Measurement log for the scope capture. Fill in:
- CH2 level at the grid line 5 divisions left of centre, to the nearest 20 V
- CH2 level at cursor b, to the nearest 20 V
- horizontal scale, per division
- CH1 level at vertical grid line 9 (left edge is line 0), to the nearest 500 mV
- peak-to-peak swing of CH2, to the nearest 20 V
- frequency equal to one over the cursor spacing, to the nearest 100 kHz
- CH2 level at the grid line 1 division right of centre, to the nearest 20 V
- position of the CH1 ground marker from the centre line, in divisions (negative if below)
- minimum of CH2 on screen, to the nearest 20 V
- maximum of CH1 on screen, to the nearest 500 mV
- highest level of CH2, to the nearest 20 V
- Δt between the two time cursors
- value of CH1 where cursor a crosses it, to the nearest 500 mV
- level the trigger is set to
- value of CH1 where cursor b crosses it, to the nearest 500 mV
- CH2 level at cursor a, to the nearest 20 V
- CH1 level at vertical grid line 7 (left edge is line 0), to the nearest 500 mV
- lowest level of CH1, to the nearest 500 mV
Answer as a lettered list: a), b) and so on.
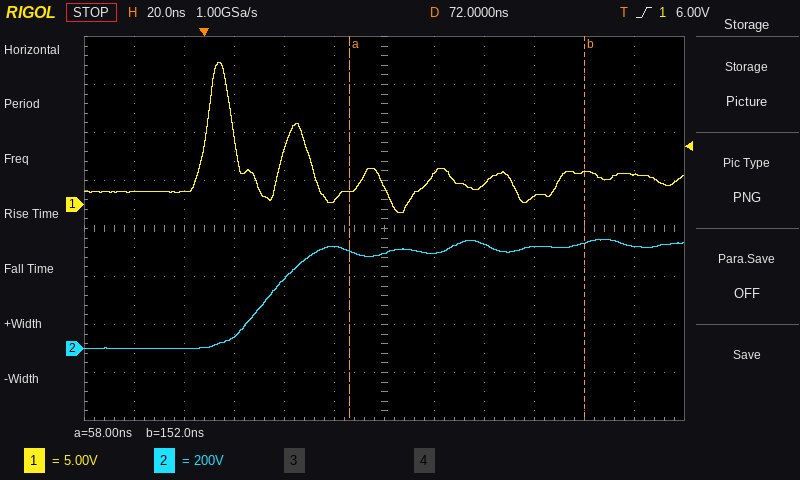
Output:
a) 0 V
b) 440 V
c) 20 ns
d) 1.0 V
e) 460 V
f) 10.6 MHz
g) 400 V
h) +0.5 div
i) 0 V
j) 15.0 V
k) 460 V
l) 94 ns
m) 1.5 V
n) 6.00 V
o) 3.5 V
p) 400 V
q) 3.0 V
r) -1.0 V
